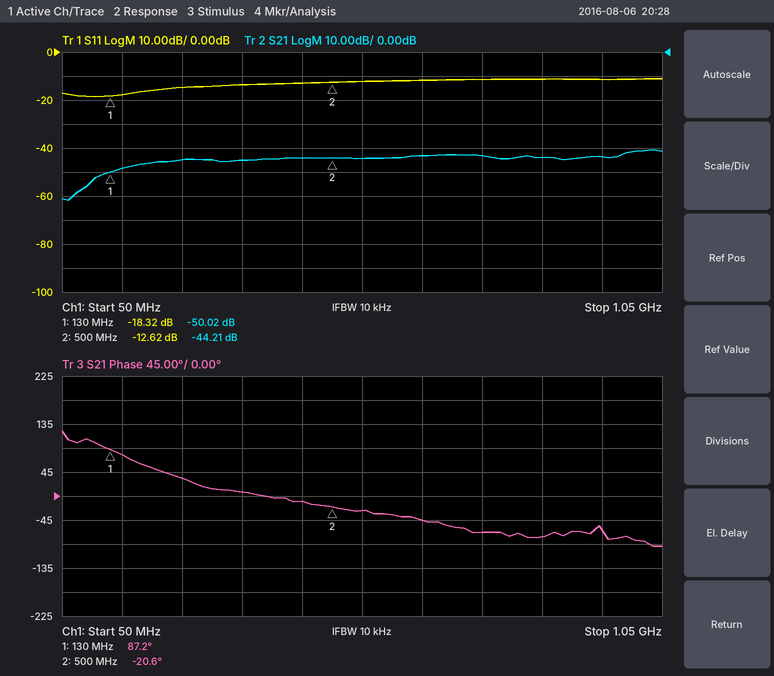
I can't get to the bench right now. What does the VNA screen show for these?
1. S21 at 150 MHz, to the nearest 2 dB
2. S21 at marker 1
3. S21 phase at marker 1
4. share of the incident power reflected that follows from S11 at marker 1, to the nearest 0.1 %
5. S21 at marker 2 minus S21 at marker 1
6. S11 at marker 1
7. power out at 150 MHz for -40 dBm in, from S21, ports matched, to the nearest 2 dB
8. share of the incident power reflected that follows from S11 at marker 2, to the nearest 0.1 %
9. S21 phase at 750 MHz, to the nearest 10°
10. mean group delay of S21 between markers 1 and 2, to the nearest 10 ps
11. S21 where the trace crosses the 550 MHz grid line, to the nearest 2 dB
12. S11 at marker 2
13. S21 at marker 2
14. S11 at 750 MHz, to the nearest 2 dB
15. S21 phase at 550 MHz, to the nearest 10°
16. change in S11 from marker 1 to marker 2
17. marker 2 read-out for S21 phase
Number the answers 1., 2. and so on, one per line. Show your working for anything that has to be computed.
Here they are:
1. -48 dB
2. -50.02 dB
3. 87.2°
4. 10^(-18.32/10) ≈ 1.5 %
5. -44.21 − (-50.02) = 5.81 dB
6. -18.32 dB
7. -40 dBm + (-48 dB) = -88 dBm
8. 10^(-12.62/10) ≈ 5.5 %
9. -70°
10. −(-20.6° − (87.2°))/(360° × 370 MHz) ≈ 809 ps, so 810 ps to the nearest 10 ps
11. -44 dB
12. -12.62 dB
13. -44.21 dB
14. -12 dB
15. -30°
16. -12.62 − (-18.32) = 5.70 dB
17. -20.6°
